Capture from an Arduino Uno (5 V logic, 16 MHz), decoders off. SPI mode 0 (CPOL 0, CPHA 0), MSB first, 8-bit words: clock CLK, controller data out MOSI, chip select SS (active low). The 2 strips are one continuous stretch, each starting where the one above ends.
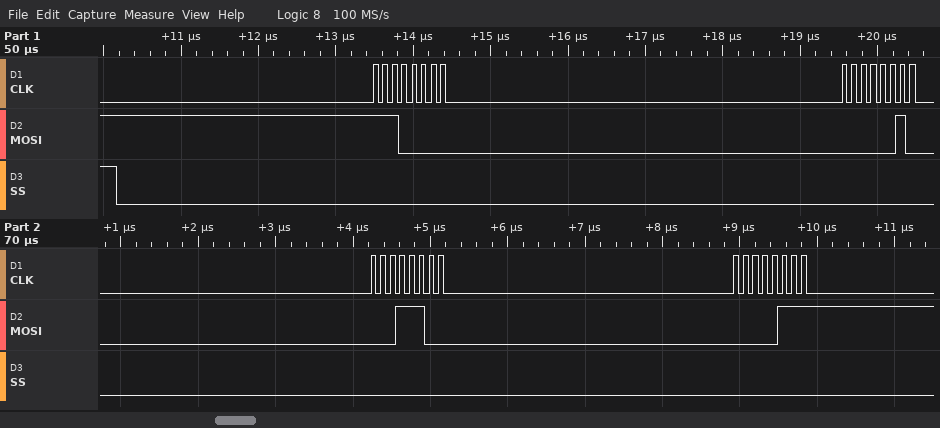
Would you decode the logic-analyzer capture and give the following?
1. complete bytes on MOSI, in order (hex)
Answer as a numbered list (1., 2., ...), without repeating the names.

1. E0 02 1C 07
